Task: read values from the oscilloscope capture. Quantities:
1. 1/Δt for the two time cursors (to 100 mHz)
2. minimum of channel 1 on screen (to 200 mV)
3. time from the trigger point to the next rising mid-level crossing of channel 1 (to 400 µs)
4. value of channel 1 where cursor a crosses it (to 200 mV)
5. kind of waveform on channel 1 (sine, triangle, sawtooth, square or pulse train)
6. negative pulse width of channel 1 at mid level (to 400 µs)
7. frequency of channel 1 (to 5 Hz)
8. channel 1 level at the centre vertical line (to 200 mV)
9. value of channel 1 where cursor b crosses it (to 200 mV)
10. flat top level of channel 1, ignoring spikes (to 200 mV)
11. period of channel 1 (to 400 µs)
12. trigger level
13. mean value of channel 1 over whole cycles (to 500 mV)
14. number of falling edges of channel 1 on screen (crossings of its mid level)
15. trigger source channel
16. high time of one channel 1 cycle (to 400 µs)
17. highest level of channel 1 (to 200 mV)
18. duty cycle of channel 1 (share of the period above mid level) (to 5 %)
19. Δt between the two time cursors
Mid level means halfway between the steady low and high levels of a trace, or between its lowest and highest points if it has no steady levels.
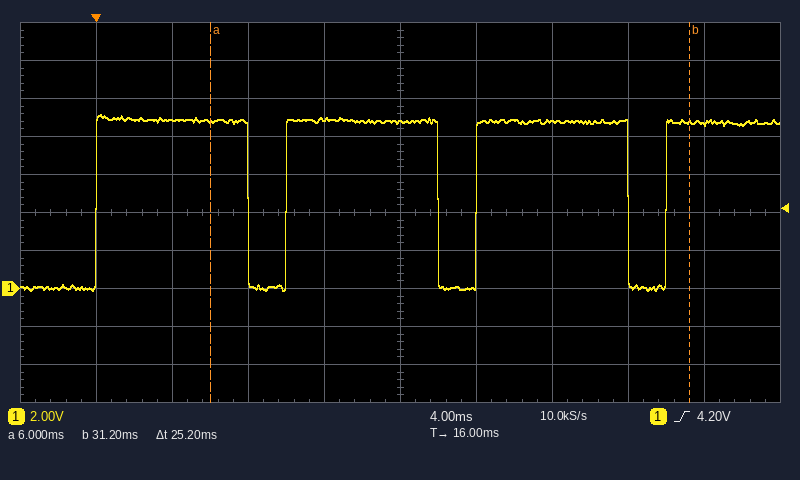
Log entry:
39.7 Hz
-200 mV
10.0 ms
8.8 V
pulse train
2.0 ms
100 Hz
8.8 V
8.8 V
8.8 V
10.0 ms
4.20 V
7.0 V
3
channel 1
8.0 ms
9.2 V
80 %
25.2 ms
